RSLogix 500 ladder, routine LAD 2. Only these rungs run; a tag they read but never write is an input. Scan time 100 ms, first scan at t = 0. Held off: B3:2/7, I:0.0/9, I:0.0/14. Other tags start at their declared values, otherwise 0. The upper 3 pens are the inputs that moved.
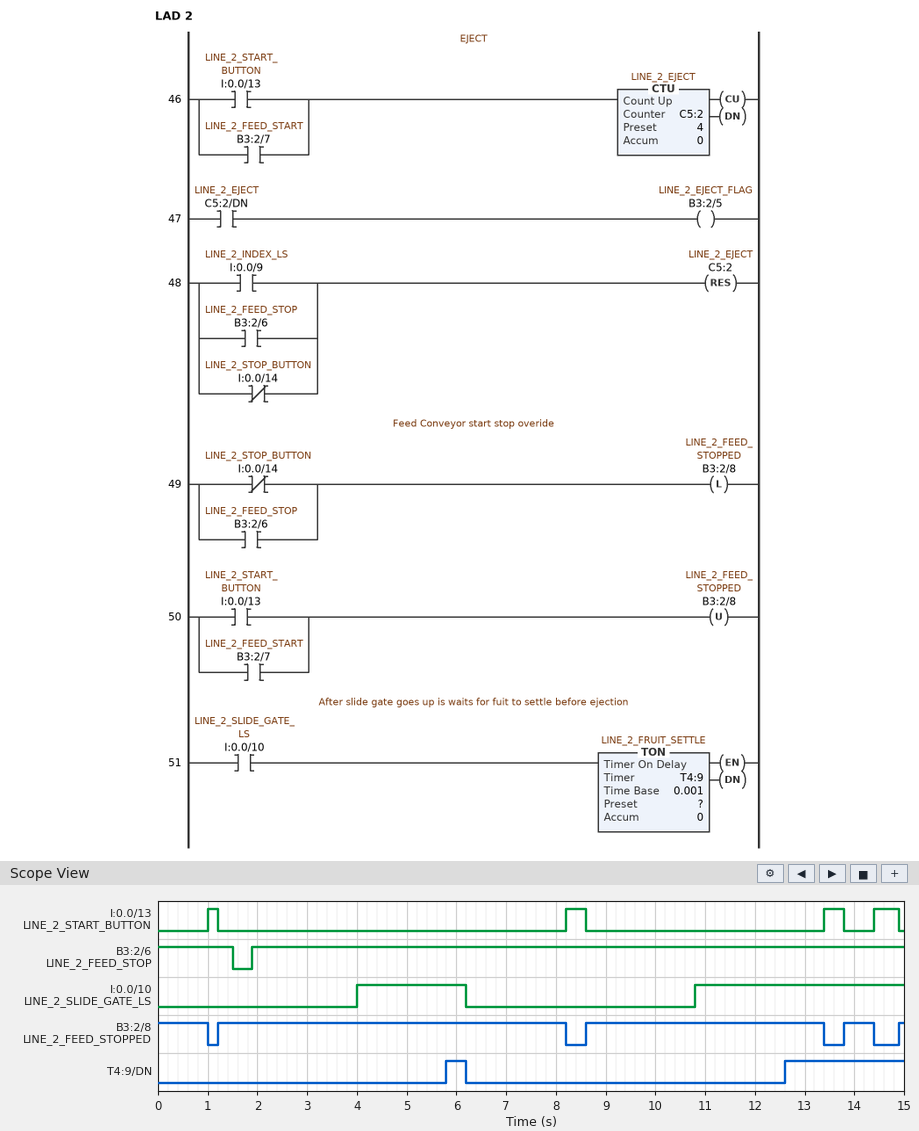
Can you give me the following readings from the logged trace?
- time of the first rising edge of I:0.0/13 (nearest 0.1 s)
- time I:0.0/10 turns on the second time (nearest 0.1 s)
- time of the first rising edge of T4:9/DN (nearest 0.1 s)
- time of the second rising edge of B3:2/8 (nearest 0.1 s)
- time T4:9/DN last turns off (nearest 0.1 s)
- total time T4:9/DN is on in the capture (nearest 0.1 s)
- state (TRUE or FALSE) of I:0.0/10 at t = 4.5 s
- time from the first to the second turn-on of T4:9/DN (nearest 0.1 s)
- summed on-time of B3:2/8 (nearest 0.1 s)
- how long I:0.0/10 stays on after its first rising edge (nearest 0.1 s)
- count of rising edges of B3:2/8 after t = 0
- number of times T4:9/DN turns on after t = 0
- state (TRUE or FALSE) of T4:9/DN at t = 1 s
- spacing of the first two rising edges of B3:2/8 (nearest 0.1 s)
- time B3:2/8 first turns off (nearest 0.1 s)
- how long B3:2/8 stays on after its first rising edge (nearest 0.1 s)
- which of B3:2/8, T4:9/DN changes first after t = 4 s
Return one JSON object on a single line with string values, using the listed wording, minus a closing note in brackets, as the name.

{"time of the first rising edge of I:0.0/13": "1.0 s", "time I:0.0/10 turns on the second time": "10.8 s", "time of the first rising edge of T4:9/DN": "5.8 s", "time of the second rising edge of B3:2/8": "8.6 s", "time T4:9/DN last turns off": "6.2 s", "total time T4:9/DN is on in the capture": "2.8 s", "state (TRUE or FALSE) of I:0.0/10 at t = 4.5 s": "TRUE", "time from the first to the second turn-on of T4:9/DN": "6.8 s", "summed on-time of B3:2/8": "13.5 s", "how long I:0.0/10 stays on after its first rising edge": "2.2 s", "count of rising edges of B3:2/8 after t = 0": "4", "number of times T4:9/DN turns on after t = 0": "2", "state (TRUE or FALSE) of T4:9/DN at t = 1 s": "FALSE", "spacing of the first two rising edges of B3:2/8": "7.4 s", "time B3:2/8 first turns off": "1.0 s", "how long B3:2/8 stays on after its first rising edge": "7.0 s", "which of B3:2/8, T4:9/DN changes first after t = 4 s": "T4:9/DN"}
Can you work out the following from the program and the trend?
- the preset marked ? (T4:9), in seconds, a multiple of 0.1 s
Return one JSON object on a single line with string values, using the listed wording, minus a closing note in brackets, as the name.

{"the preset marked ? (T4:9), in seconds, a multiple of 0.1 s": "1.8 s"}
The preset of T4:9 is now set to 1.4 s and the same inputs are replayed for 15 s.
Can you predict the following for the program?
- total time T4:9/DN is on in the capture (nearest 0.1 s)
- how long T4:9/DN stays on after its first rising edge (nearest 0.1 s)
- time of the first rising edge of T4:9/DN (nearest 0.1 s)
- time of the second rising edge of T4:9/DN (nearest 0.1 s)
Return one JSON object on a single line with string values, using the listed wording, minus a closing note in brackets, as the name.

{"total time T4:9/DN is on in the capture": "3.6 s", "how long T4:9/DN stays on after its first rising edge": "0.8 s", "time of the first rising edge of T4:9/DN": "5.4 s", "time of the second rising edge of T4:9/DN": "12.2 s"}
